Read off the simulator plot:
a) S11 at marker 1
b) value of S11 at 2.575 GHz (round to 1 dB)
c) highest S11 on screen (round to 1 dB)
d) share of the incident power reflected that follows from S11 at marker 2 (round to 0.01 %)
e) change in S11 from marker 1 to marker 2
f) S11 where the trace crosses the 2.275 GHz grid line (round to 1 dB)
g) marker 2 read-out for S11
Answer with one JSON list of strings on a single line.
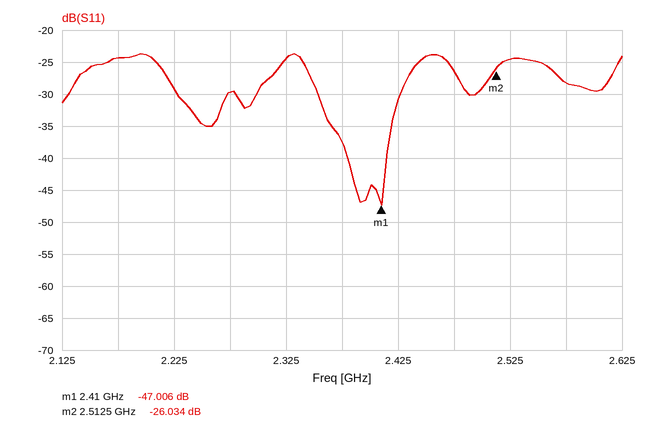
["-47.006 dB", "-28 dB", "-24 dB", "0.25 %", "20.972 dB", "-30 dB", "-26.034 dB"]
